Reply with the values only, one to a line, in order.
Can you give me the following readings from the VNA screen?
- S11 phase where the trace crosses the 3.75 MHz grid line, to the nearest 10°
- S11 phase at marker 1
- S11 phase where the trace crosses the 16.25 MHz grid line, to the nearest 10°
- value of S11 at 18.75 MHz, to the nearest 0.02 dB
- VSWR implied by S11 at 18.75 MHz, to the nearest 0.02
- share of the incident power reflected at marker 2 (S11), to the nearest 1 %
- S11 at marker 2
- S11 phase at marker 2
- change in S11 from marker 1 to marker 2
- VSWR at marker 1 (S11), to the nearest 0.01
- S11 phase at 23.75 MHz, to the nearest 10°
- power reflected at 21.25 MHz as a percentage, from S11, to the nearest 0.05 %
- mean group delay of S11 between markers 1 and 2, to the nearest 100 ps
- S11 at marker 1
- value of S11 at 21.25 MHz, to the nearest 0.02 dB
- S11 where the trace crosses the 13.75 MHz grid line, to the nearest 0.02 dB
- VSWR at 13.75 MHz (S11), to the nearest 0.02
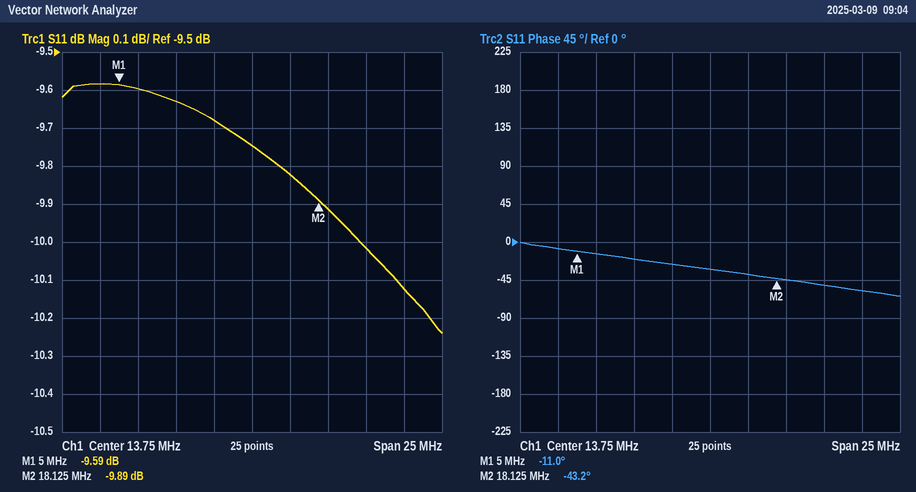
-10°
-11.0°
-40°
-9.92 dB
1.94
10 %
-9.89 dB
-43.2°
-0.30 dB
1.99
-60°
9.95 %
6.8 ns
-9.59 dB
-10.02 dB
-9.74 dB
1.96
